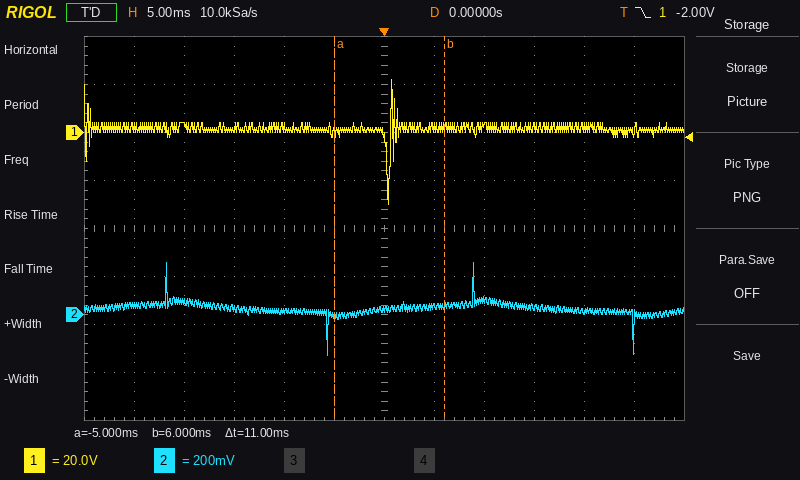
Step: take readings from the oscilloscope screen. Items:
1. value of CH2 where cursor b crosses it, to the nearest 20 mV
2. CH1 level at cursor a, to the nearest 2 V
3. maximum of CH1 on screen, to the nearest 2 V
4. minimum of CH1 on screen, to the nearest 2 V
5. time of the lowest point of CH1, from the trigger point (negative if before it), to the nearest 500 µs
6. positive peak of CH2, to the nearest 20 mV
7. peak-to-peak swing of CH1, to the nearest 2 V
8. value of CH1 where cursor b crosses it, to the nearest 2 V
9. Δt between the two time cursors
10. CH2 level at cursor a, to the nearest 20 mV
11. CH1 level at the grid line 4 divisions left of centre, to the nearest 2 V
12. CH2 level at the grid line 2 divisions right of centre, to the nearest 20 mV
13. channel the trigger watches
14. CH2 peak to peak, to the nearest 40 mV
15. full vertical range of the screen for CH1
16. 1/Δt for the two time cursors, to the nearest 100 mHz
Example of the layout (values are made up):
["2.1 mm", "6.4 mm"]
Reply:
["40 mV", "0 V", "22 V", "-30 V", "+500 µs", "220 mV", "52 V", "2 V", "11 ms", "0 mV", "2 V", "60 mV", "CH1", "400 mV", "160 V", "90.9 Hz"]
